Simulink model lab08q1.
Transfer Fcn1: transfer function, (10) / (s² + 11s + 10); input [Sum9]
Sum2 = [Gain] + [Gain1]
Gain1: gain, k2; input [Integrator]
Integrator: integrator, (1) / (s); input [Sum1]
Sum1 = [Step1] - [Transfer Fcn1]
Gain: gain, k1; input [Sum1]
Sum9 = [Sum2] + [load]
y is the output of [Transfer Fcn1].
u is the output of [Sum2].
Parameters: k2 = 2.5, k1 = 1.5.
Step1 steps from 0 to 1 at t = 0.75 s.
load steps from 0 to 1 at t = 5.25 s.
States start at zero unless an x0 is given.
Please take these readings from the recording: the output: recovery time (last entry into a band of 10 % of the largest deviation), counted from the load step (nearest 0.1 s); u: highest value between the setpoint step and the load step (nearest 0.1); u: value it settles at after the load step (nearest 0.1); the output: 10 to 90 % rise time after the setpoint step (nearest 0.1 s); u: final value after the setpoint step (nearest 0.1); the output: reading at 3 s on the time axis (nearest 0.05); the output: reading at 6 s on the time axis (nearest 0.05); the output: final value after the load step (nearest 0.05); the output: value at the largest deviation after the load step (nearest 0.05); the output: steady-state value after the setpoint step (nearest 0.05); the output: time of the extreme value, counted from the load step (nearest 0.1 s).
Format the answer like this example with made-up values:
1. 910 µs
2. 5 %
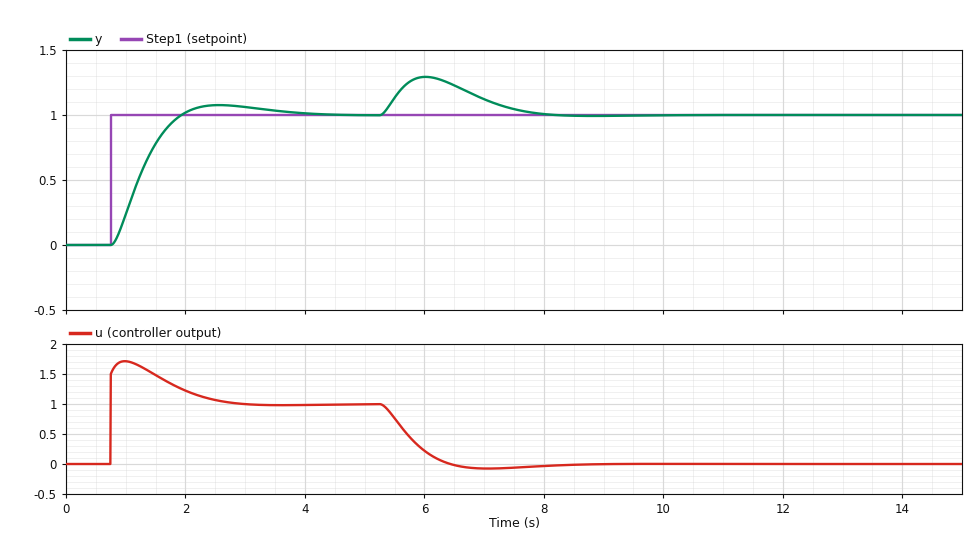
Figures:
1. 2.4 s
2. 1.7
3. 0.0
4. 0.8 s
5. 1.0
6. 1.05
7. 1.30
8. 1.00
9. 1.30
10. 1.00
11. 0.8 s
